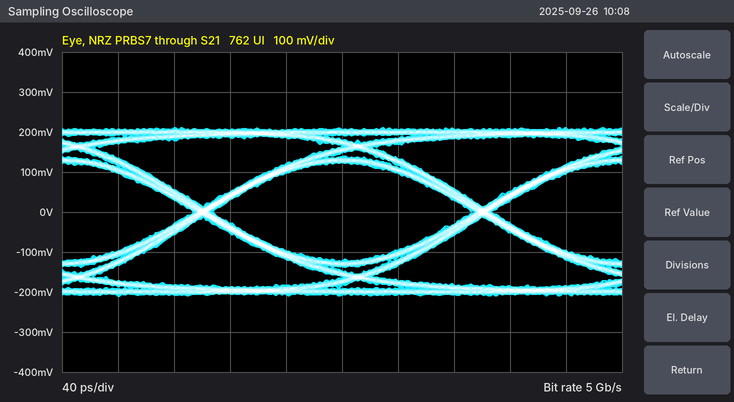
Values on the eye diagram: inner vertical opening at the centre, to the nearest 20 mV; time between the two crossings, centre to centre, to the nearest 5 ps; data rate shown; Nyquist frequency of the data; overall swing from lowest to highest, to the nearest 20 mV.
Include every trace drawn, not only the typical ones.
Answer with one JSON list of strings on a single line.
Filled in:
["240 mV", "200 ps", "5 Gb/s", "2.5 GHz", "420 mV"]
